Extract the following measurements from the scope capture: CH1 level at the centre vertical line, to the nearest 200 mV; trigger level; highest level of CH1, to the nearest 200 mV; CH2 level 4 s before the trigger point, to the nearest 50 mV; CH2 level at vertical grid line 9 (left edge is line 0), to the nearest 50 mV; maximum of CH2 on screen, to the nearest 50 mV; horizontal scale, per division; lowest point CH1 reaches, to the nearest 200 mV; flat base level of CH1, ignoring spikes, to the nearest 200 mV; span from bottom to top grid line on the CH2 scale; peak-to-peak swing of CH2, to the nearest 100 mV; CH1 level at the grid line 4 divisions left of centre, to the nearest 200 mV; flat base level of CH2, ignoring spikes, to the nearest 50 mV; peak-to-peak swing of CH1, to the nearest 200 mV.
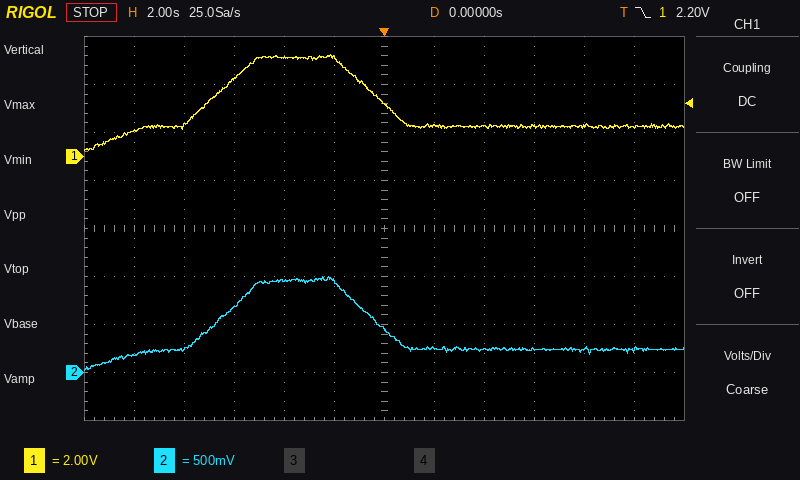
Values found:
2.2 V
2.20 V
4.2 V
950 mV
250 mV
1.00 V
2 s
200 mV
1.2 V
4 V
1.00 V
1.2 V
250 mV
4.0 V
